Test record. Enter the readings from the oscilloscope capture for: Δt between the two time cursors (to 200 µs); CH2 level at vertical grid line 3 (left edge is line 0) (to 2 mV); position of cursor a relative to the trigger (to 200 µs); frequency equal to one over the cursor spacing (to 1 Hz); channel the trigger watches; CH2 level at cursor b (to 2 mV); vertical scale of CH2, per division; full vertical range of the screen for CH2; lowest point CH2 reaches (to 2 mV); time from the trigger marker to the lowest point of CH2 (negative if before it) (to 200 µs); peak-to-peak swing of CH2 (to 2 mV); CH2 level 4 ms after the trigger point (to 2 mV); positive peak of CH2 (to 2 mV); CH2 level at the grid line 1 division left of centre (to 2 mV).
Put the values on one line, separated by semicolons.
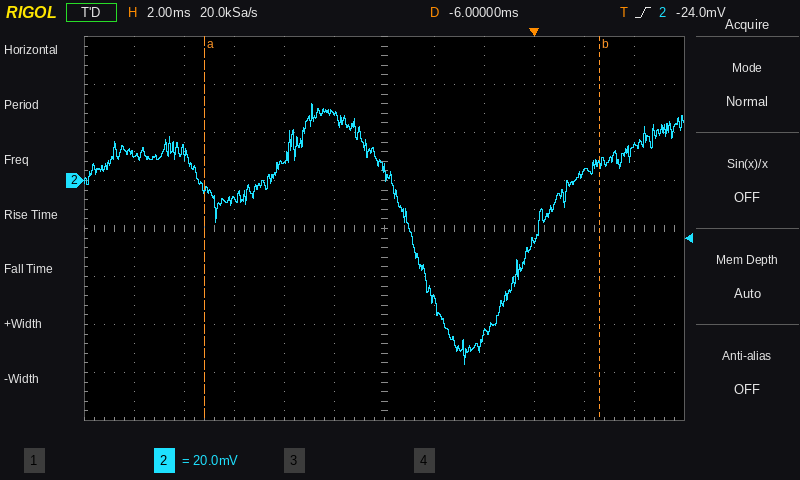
15.8 ms; -8 mV; -13.2 ms; 63 Hz; CH2; 8 mV; 20 mV; 160 mV; -76 mV; -2.8 ms; 108 mV; 14 mV; 32 mV; 28 mV
